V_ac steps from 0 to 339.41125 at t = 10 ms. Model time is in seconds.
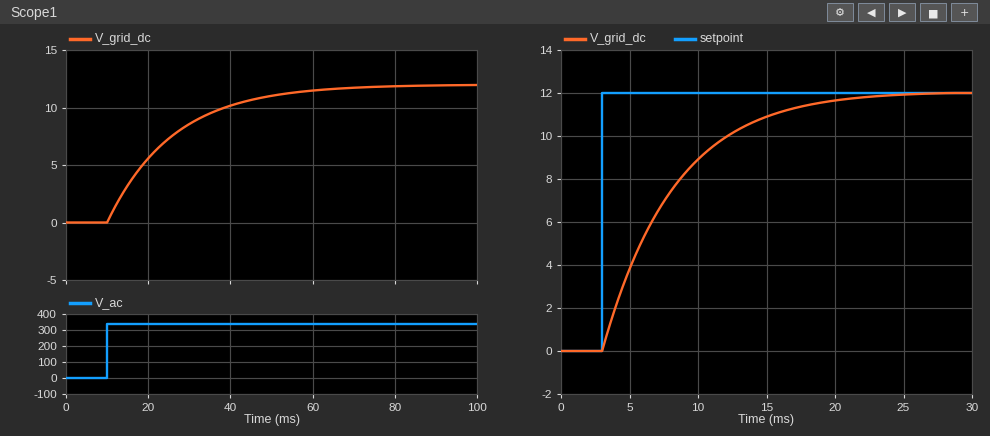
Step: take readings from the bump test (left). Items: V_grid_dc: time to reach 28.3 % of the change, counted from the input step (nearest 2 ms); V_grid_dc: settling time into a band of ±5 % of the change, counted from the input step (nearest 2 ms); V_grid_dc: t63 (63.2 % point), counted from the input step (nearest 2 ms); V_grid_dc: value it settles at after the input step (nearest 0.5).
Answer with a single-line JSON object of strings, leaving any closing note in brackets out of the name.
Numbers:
{"V_grid_dc: time to reach 28.3 % of the change, counted from the input step": "6 ms", "V_grid_dc: settling time into a band of ±5 % of the change, counted from the input step": "48 ms", "V_grid_dc: t63 (63.2 % point), counted from the input step": "16 ms", "V_grid_dc: value it settles at after the input step": "12.0"}
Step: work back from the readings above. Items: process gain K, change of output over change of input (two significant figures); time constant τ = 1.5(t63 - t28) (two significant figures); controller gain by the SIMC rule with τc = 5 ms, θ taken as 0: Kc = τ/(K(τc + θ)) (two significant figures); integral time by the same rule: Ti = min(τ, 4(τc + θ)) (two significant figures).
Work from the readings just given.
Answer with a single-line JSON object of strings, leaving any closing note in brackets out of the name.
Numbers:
{"process gain K, change of output over change of input": "0.035", "time constant τ = 1.5(t63 - t28)": "15 ms", "controller gain by the SIMC rule with τc = 5 ms, θ taken as 0: Kc = τ/(K(τc + θ))": "86", "integral time by the same rule: Ti = min(τ, 4(τc + θ))": "15 ms"}
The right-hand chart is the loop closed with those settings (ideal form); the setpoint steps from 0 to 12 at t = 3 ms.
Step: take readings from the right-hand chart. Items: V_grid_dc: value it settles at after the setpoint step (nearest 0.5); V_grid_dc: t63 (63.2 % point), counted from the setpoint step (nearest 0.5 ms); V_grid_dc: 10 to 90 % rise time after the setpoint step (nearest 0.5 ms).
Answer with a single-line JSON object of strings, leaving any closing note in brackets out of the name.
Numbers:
{"V_grid_dc: value it settles at after the setpoint step": "12.0", "V_grid_dc: t63 (63.2 % point), counted from the setpoint step": "5.0 ms", "V_grid_dc: 10 to 90 % rise time after the setpoint step": "11.0 ms"}
